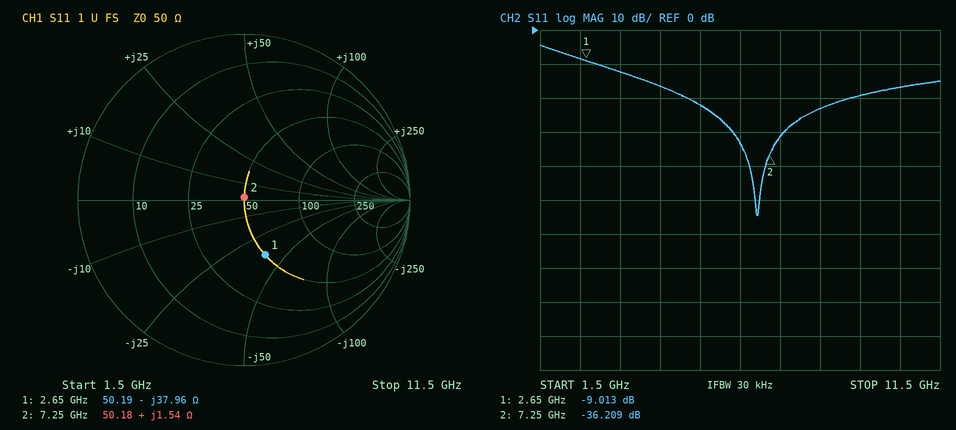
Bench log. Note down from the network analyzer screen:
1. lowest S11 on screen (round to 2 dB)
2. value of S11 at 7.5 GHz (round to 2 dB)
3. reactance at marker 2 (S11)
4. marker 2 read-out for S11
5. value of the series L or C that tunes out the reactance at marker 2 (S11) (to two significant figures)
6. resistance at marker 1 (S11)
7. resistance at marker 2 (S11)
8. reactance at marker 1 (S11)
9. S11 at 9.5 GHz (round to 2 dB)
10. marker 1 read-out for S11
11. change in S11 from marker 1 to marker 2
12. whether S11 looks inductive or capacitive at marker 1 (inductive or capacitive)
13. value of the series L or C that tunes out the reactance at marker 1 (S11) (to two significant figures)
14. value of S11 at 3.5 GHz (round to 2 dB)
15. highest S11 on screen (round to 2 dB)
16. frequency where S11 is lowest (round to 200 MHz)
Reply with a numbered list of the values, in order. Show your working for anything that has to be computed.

1. -54 dB
2. -32 dB
3. +1.54 Ω
4. -36.209 dB
5. C = 1/(2π × 7.25 GHz × 1.54 Ω) ≈ 14 pF
6. 50.19 Ω
7. 50.18 Ω
8. -37.96 Ω
9. -20 dB
10. -9.013 dB
11. -36.209 − (-9.013) = -27.196 dB
12. capacitive
13. L = 37.96 Ω/(2π × 2.65 GHz) ≈ 2.3 nH
14. -12 dB
15. -4 dB
16. 7.0 GHz
